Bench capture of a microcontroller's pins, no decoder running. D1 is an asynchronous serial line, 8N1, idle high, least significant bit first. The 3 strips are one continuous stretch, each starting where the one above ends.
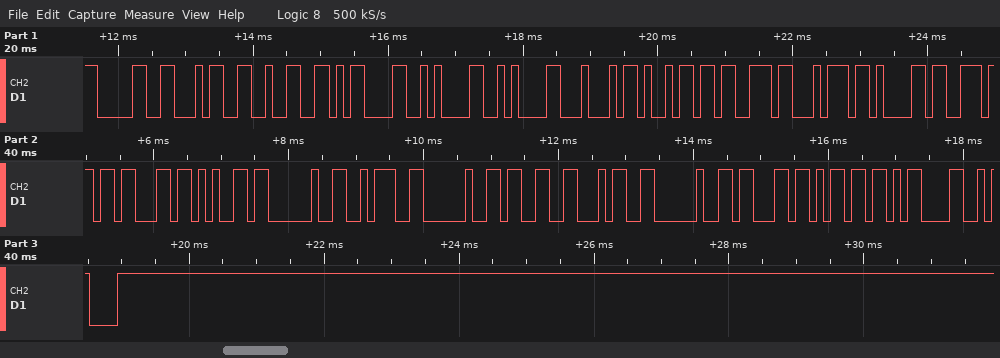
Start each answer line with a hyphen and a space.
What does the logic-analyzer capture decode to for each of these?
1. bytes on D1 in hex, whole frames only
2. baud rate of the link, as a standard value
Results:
- 30 34 32 0D 0A 0A 44 69 73 74 61 6E 63 65 20 3A 20 33 34 20 63 6D 0D 0A
- 9600 baud
